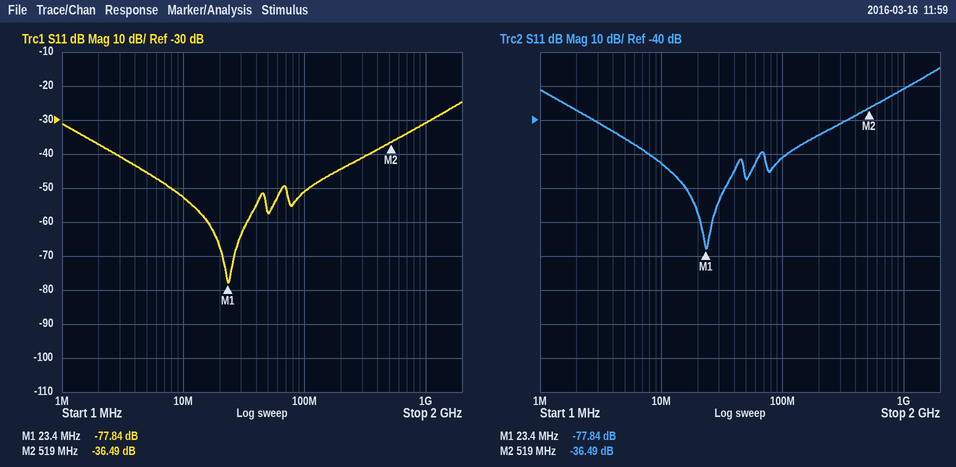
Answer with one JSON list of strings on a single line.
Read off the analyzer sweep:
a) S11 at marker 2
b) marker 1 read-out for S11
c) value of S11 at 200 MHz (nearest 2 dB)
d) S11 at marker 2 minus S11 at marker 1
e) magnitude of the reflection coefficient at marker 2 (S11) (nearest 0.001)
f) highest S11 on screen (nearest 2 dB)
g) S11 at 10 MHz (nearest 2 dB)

["-36.49 dB", "-77.84 dB", "-44 dB", "41.35 dB", "0.015", "-24 dB", "-52 dB"]
